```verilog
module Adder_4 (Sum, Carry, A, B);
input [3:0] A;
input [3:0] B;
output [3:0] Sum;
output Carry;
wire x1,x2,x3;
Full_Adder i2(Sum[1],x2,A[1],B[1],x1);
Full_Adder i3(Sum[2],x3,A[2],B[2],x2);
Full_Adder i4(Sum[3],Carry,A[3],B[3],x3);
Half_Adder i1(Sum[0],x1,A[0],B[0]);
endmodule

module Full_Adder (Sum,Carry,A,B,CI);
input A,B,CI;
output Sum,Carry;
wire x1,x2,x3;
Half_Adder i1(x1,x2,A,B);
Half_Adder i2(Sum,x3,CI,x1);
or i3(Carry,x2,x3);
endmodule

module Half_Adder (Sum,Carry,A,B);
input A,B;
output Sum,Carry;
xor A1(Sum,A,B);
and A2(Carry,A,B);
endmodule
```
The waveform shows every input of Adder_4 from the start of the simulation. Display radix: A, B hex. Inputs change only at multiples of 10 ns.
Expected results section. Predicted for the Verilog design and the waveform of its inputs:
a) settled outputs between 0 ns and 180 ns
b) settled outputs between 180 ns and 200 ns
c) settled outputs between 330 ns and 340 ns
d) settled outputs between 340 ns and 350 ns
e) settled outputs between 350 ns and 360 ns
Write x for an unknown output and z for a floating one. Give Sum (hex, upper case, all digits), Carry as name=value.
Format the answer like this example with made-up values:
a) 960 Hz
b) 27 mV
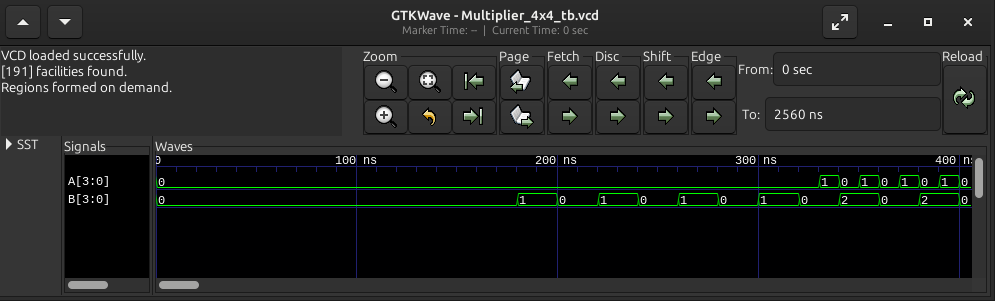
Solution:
a) Sum=0, Carry=0
b) Sum=1, Carry=0
c) Sum=1, Carry=0
d) Sum=2, Carry=0
e) Sum=3, Carry=0
